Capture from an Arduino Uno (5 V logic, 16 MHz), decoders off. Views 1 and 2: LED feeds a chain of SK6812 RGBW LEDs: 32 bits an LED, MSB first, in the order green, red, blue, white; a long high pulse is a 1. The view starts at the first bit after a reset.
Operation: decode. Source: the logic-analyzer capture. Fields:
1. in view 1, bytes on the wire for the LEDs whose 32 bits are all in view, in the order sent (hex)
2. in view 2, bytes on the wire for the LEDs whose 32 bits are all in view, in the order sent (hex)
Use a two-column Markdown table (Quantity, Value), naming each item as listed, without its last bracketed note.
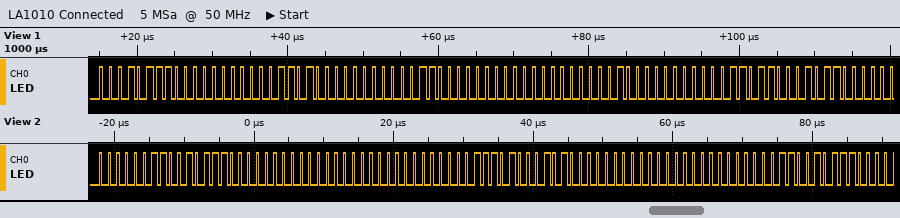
| Quantity | Value |
|---|---|
| in view 1, bytes on the wire for the LEDs whose 32 bits are all in view, in the order sent | 17 00 1A 00 30 00 01 00 |
| in view 2, bytes on the wire for the LEDs whose 32 bits are all in view, in the order sent | 03 2E 00 00 00 1D 14 00 |
